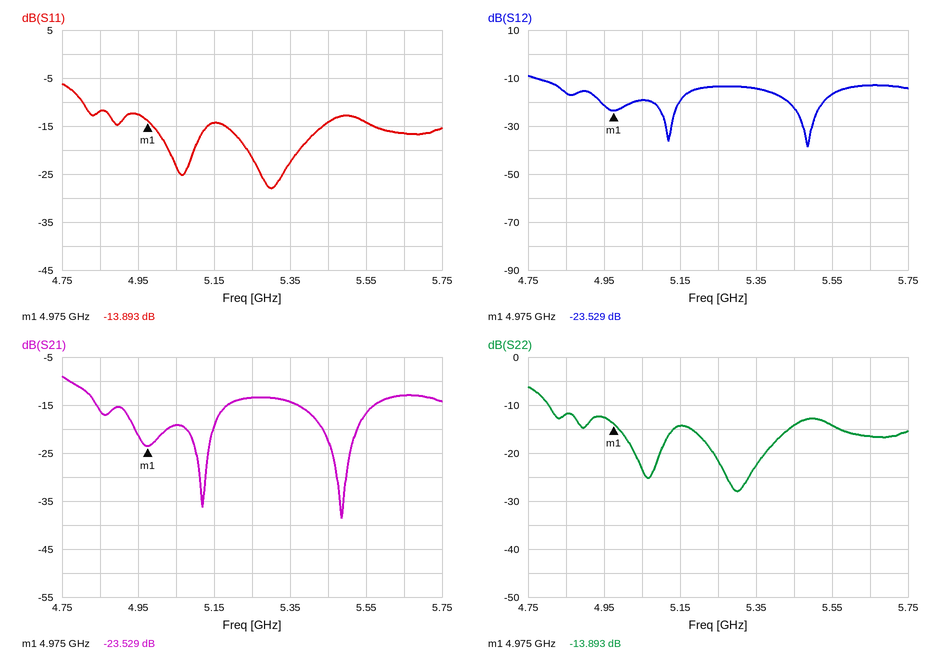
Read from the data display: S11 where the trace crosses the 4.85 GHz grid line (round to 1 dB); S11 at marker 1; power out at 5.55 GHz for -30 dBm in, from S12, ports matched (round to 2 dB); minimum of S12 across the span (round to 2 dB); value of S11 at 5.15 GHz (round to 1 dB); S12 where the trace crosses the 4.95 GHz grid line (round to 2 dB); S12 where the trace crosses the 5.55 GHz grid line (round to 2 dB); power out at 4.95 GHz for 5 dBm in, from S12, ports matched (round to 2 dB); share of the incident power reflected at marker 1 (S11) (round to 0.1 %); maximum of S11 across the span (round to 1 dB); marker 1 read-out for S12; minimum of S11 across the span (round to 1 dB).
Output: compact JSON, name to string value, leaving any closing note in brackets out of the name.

{"S11 where the trace crosses the 4.85 GHz grid line": "-12 dB", "S11 at marker 1": "-13.893 dB", "power out at 5.55 GHz for -30 dBm in, from S12, ports matched": "-46 dBm", "minimum of S12 across the span": "-38 dB", "value of S11 at 5.15 GHz": "-14 dB", "S12 where the trace crosses the 4.95 GHz grid line": "-22 dB", "S12 where the trace crosses the 5.55 GHz grid line": "-16 dB", "power out at 4.95 GHz for 5 dBm in, from S12, ports matched": "-16 dBm", "share of the incident power reflected at marker 1 (S11)": "4.1 %", "maximum of S11 across the span": "-6 dB", "marker 1 read-out for S12": "-23.529 dB", "minimum of S11 across the span": "-28 dB"}
